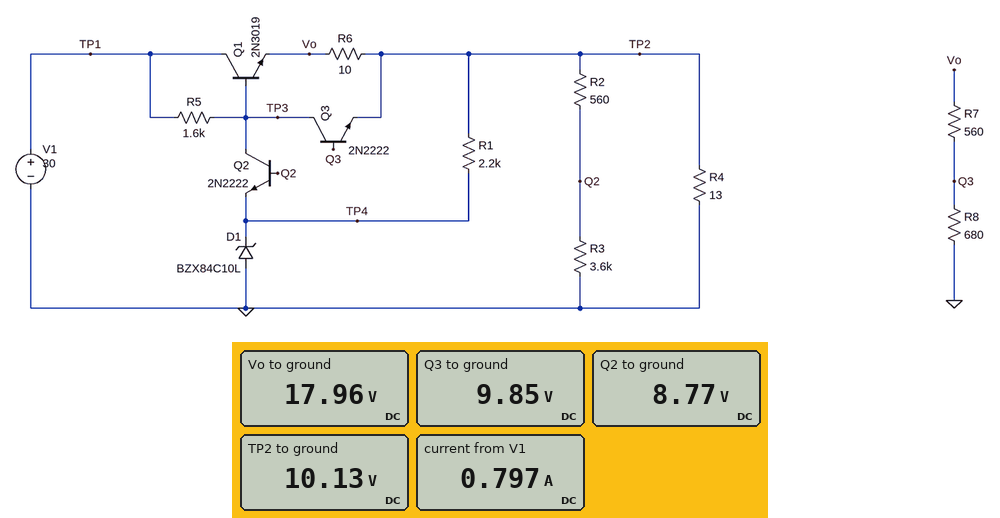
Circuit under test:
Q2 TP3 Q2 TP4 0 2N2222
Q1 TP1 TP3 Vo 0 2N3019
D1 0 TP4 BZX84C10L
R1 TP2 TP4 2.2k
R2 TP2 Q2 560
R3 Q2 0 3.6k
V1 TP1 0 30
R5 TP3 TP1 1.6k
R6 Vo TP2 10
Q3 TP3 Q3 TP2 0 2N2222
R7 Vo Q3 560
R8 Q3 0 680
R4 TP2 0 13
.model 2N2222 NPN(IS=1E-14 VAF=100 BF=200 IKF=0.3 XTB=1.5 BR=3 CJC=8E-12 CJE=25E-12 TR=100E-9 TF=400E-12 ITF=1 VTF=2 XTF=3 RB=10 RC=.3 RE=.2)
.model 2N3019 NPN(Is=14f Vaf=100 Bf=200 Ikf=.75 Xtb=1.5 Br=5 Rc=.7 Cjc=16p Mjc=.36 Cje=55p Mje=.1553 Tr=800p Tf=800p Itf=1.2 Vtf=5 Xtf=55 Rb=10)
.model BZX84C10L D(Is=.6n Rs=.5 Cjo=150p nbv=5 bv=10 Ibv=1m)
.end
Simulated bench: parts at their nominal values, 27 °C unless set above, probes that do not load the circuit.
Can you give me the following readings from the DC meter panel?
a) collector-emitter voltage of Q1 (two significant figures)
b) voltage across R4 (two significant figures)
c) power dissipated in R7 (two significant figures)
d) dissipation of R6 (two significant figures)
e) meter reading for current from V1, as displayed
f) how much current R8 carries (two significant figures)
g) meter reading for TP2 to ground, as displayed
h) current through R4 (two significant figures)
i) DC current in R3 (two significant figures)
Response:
12 V
10 V
120 mW
6.1 W
0.797 A
14 mA
10.13 V
780 mA
2.4 mA
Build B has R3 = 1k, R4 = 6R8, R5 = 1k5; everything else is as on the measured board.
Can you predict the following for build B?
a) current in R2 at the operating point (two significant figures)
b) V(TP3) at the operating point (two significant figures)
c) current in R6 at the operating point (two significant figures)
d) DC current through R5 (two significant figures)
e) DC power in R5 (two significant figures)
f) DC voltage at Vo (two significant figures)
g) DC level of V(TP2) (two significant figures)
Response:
1.5 mA
6.4 V
330 mA
16 mA
370 mW
5.6 V
2.3 V
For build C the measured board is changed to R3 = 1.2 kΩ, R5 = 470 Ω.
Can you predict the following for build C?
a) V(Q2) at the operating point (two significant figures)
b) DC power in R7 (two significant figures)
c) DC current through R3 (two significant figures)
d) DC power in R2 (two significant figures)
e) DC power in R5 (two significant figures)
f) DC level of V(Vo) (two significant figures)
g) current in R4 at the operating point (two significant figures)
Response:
9.1 V
200 mW
7.6 mA
32 mW
62 mW
24 V
1.0 A
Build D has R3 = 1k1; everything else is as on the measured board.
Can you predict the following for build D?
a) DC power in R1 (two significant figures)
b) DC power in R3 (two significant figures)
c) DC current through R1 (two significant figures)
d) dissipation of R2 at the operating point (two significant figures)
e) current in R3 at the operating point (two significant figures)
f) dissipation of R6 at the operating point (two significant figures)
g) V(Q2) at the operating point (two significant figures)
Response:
53 µW
41 mW
160 µA
21 mW
6.1 mA
6.1 W
6.7 V
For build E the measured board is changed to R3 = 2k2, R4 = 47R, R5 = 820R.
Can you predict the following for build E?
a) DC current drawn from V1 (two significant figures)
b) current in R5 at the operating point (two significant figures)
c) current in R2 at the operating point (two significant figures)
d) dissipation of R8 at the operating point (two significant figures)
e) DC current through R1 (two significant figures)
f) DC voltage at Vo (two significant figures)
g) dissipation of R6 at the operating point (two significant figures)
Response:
330 mA
15 mA
5.1 mA
130 mW
1.6 mA
17 V
920 mW
